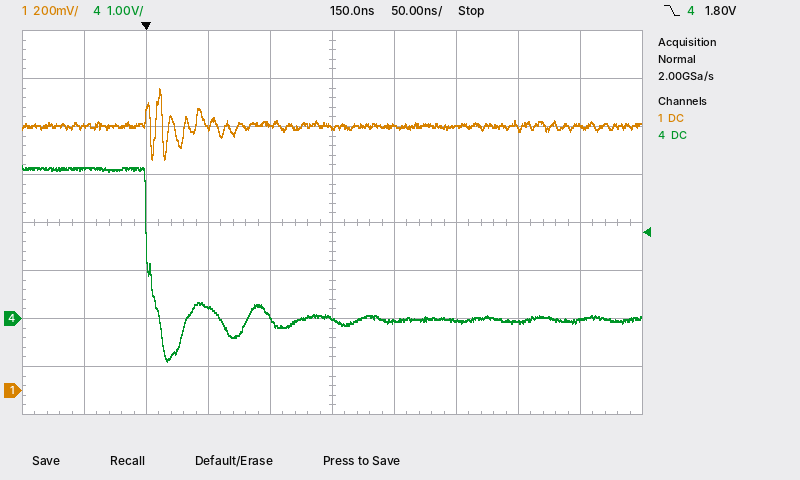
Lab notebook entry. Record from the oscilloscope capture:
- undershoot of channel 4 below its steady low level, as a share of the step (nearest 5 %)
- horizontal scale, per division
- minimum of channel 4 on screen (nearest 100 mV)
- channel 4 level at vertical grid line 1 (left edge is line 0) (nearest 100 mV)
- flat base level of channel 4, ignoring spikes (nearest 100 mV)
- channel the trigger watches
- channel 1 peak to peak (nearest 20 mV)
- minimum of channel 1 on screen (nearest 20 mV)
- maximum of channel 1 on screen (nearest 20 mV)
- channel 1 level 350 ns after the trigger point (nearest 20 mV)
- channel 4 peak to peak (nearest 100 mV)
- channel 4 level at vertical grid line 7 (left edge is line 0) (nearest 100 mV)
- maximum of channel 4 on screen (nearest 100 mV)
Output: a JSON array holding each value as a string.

["30 %", "50 ns", "-900 mV", "3.1 V", "0.0 V", "channel 4", "300 mV", "960 mV", "1.26 V", "1.10 V", "4.1 V", "0.0 V", "3.2 V"]
